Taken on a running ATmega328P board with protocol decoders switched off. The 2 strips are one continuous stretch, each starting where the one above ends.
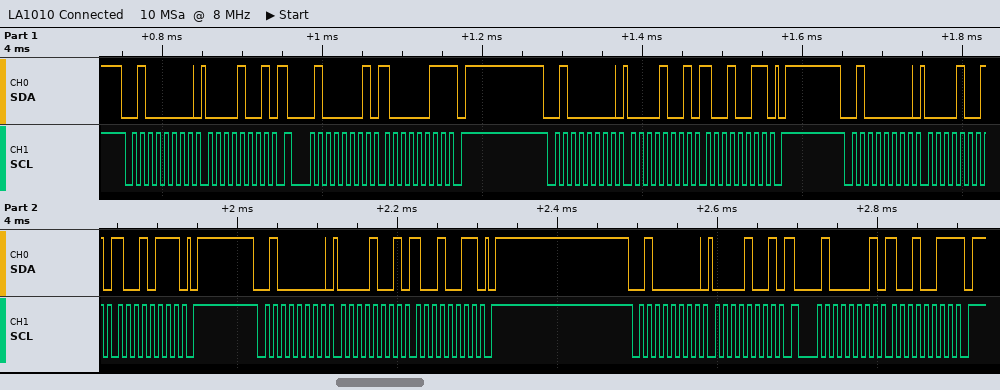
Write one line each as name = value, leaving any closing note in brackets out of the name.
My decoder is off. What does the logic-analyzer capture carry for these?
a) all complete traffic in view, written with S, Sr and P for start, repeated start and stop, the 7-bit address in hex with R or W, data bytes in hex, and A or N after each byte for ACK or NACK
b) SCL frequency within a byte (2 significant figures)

all complete traffic in view, written with S, Sr and P for start, repeated start and stop, the 7-bit address in hex with R or W, data bytes in hex, and A or N after each byte for ACK or NACK = S 20W A 09 A Sr 20R A 83 N P S 20W A 09 A 93 A P S 20W A 09 A 97 A P S 20W A 09 A 93 A P S 20W A 09 A Sr 20R A 93 N P
SCL frequency within a byte = 100 kHz
